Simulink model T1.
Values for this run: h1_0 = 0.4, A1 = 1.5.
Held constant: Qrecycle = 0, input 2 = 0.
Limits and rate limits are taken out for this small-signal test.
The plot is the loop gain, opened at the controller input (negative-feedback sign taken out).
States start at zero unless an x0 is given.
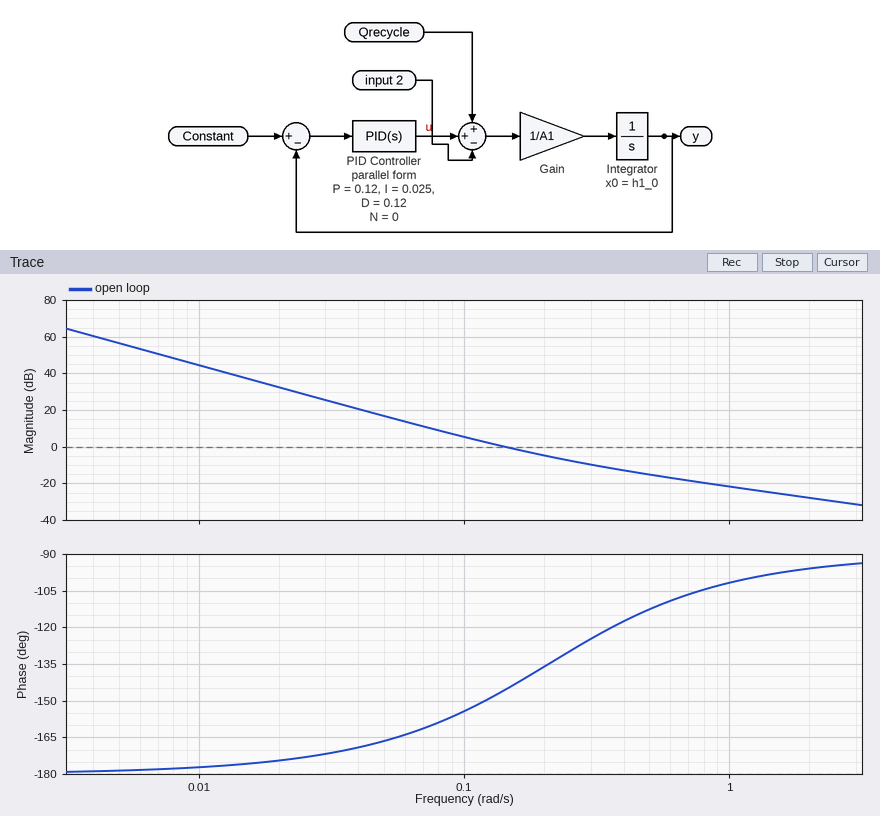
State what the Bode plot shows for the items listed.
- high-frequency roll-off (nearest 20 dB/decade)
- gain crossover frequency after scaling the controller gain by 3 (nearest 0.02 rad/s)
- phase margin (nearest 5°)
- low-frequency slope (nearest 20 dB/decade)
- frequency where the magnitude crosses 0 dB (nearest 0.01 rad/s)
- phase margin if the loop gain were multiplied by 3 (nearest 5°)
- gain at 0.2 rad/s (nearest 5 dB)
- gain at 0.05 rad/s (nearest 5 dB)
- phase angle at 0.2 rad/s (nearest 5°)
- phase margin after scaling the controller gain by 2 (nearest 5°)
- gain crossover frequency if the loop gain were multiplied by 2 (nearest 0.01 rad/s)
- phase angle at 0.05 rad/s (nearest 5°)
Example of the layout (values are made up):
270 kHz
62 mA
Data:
-20 dB/decade
0.30 rad/s
35°
-40 dB/decade
0.14 rad/s
55°
-5 dB
15 dB
-135°
45°
0.22 rad/s
-165°
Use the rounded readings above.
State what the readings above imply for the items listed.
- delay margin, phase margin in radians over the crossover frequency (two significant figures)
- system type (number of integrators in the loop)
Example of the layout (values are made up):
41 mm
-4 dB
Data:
4.4 s
2
